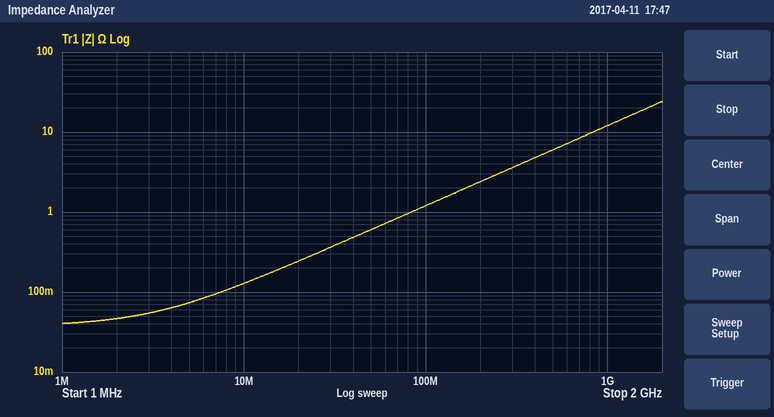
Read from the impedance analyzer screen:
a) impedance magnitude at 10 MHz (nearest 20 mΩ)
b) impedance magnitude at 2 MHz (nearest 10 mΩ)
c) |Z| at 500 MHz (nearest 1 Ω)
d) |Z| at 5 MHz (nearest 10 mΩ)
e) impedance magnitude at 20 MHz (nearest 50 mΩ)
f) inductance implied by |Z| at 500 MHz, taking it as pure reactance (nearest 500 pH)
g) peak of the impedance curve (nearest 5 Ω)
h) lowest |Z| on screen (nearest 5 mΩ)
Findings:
120 mΩ
50 mΩ
6 Ω
70 mΩ
250 mΩ
2.0 nH
25 Ω
40 mΩ
